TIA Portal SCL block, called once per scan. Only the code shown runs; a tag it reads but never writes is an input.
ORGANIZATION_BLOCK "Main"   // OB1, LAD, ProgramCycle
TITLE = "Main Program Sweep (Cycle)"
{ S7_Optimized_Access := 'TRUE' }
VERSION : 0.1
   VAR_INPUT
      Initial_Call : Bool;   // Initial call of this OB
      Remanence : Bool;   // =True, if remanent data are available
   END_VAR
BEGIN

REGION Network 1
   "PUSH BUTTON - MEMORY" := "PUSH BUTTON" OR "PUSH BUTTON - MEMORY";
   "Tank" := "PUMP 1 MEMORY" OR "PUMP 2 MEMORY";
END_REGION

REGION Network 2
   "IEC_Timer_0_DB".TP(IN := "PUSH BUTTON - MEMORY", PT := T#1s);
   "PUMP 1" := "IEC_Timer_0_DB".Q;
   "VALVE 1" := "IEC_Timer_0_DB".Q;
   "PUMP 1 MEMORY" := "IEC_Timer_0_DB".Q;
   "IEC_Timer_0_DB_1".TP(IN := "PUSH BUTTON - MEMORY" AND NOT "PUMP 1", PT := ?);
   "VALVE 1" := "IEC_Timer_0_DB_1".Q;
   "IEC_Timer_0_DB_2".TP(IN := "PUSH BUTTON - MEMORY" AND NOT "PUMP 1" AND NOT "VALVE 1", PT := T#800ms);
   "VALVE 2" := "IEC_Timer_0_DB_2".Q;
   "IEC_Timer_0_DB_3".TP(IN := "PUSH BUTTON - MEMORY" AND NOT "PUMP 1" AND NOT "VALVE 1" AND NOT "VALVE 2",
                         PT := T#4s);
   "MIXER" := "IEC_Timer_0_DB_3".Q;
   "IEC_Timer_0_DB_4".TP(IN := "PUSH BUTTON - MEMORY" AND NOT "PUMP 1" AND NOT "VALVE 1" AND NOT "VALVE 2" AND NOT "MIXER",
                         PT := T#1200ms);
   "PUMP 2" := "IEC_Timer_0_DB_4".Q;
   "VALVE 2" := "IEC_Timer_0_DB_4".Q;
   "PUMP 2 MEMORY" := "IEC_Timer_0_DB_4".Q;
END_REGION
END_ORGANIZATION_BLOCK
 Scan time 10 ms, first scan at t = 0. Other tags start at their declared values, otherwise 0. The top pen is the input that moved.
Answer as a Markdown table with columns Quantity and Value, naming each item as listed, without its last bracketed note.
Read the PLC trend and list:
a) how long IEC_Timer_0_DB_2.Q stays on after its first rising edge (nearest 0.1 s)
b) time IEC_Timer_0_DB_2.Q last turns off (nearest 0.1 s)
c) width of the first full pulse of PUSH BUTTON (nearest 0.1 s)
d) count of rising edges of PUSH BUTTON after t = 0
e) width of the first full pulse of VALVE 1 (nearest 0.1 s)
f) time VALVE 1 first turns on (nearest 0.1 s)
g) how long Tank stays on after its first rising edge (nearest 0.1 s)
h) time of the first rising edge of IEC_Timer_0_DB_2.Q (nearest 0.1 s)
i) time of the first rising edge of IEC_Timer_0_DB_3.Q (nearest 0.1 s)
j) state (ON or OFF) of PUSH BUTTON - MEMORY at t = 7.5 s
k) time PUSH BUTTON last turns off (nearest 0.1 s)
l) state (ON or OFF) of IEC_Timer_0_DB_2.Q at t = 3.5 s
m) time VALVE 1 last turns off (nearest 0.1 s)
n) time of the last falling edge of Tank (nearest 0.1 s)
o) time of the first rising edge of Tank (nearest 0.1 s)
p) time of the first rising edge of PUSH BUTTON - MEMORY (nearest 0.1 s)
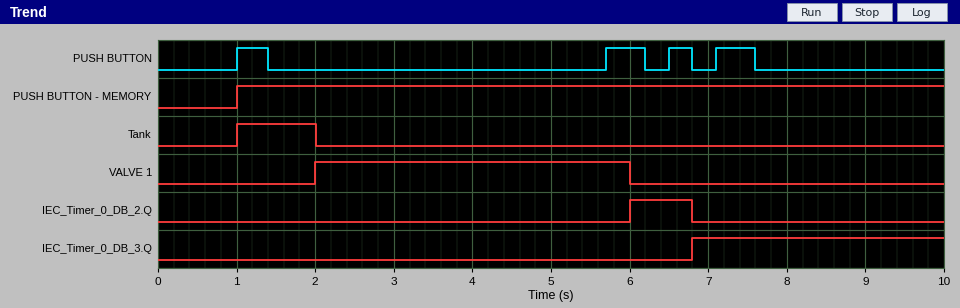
| Quantity | Value |
|---|---|
| how long IEC_Timer_0_DB_2.Q stays on after its first rising edge | 0.8 s |
| time IEC_Timer_0_DB_2.Q last turns off | 6.8 s |
| width of the first full pulse of PUSH BUTTON | 0.4 s |
| count of rising edges of PUSH BUTTON after t = 0 | 4 |
| width of the first full pulse of VALVE 1 | 4.0 s |
| time VALVE 1 first turns on | 2.0 s |
| how long Tank stays on after its first rising edge | 1.0 s |
| time of the first rising edge of IEC_Timer_0_DB_2.Q | 6.0 s |
| time of the first rising edge of IEC_Timer_0_DB_3.Q | 6.8 s |
| state (ON or OFF) of PUSH BUTTON - MEMORY at t = 7.5 s | ON |
| time PUSH BUTTON last turns off | 7.6 s |
| state (ON or OFF) of IEC_Timer_0_DB_2.Q at t = 3.5 s | OFF |
| time VALVE 1 last turns off | 6.0 s |
| time of the last falling edge of Tank | 2.0 s |
| time of the first rising edge of Tank | 1.0 s |
| time of the first rising edge of PUSH BUTTON - MEMORY | 1.0 s |
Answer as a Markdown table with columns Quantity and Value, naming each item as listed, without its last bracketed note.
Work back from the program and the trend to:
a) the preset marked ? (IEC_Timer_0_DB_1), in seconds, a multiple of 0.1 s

| Quantity | Value |
|---|---|
| the preset marked ? (IEC_Timer_0_DB_1), in seconds, a multiple of 0.1 s | 4.0 s |
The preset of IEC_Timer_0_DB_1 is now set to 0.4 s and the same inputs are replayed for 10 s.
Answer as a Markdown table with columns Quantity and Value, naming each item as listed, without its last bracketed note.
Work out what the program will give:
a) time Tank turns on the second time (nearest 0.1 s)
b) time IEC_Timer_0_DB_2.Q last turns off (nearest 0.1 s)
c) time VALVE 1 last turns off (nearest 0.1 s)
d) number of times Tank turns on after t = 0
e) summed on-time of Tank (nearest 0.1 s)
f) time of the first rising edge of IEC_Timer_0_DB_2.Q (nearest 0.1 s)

| Quantity | Value |
|---|---|
| time Tank turns on the second time | 7.2 s |
| time IEC_Timer_0_DB_2.Q last turns off | 3.2 s |
| time VALVE 1 last turns off | 2.4 s |
| number of times Tank turns on after t = 0 | 2 |
| summed on-time of Tank | 2.2 s |
| time of the first rising edge of IEC_Timer_0_DB_2.Q | 2.4 s |
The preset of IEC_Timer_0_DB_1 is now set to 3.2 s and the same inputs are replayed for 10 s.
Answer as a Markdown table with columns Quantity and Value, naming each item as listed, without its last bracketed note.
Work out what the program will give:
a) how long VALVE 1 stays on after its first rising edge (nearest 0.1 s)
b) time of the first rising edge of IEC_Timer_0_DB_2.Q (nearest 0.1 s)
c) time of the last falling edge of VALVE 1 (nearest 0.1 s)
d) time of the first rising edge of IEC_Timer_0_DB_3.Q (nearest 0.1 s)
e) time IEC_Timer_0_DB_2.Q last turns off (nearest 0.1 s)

| Quantity | Value |
|---|---|
| how long VALVE 1 stays on after its first rising edge | 3.2 s |
| time of the first rising edge of IEC_Timer_0_DB_2.Q | 5.2 s |
| time of the last falling edge of VALVE 1 | 5.2 s |
| time of the first rising edge of IEC_Timer_0_DB_3.Q | 6.0 s |
| time IEC_Timer_0_DB_2.Q last turns off | 6.0 s |
